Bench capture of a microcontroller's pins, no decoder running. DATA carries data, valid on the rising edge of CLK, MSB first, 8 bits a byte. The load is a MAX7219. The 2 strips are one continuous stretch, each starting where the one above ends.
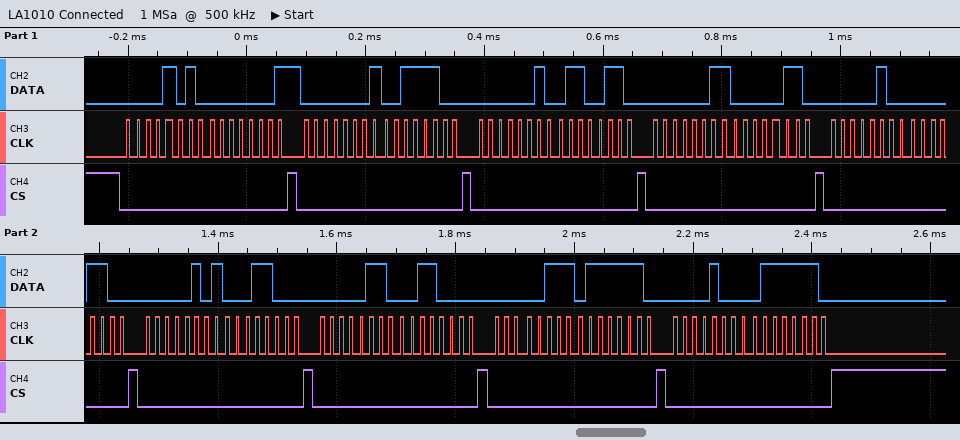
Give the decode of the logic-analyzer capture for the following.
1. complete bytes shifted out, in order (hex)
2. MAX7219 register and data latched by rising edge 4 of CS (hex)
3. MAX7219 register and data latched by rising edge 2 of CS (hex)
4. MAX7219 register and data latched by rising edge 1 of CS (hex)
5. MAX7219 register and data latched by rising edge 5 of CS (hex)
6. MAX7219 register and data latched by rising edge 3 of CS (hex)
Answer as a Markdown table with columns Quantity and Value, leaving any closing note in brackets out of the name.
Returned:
| Quantity | Value |
|---|---|
| complete bytes shifted out, in order | 0x0A 0x01 0x01 0x3C 0x02 0x66 0x03 0x06 0x04 0x0C 0x05 0x18 0x06 0x30 0x07 0x7E 0x08 0x7E |
| MAX7219 register and data latched by rising edge 4 of CS | register 0x3, data 0x06 |
| MAX7219 register and data latched by rising edge 2 of CS | register 0x1, data 0x3C |
| MAX7219 register and data latched by rising edge 1 of CS | register 0xA, data 0x01 |
| MAX7219 register and data latched by rising edge 5 of CS | register 0x4, data 0x0C |
| MAX7219 register and data latched by rising edge 3 of CS | register 0x2, data 0x66 |
